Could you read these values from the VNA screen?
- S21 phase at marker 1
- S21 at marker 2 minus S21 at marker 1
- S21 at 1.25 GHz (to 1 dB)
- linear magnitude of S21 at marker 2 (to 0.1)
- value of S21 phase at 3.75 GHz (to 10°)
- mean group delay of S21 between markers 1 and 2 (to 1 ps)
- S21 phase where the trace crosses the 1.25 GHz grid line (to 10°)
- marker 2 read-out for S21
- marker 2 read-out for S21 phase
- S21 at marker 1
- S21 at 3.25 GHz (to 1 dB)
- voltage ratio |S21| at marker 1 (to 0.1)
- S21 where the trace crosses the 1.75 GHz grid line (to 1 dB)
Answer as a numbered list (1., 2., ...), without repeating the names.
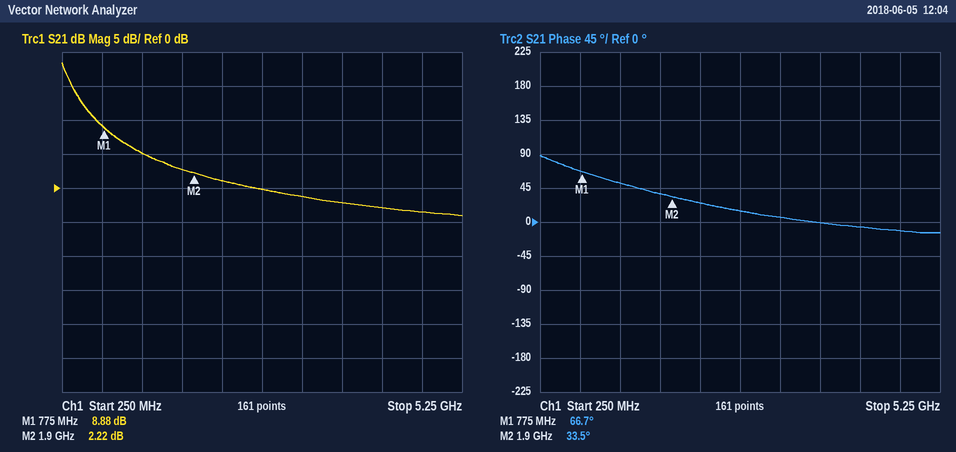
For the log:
1. 66.7°
2. -6.66 dB
3. 5 dB
4. 1.3
5. 0°
6. 82 ps
7. 50°
8. 2.22 dB
9. 33.5°
10. 8.88 dB
11. -1 dB
12. 2.8
13. 3 dB
